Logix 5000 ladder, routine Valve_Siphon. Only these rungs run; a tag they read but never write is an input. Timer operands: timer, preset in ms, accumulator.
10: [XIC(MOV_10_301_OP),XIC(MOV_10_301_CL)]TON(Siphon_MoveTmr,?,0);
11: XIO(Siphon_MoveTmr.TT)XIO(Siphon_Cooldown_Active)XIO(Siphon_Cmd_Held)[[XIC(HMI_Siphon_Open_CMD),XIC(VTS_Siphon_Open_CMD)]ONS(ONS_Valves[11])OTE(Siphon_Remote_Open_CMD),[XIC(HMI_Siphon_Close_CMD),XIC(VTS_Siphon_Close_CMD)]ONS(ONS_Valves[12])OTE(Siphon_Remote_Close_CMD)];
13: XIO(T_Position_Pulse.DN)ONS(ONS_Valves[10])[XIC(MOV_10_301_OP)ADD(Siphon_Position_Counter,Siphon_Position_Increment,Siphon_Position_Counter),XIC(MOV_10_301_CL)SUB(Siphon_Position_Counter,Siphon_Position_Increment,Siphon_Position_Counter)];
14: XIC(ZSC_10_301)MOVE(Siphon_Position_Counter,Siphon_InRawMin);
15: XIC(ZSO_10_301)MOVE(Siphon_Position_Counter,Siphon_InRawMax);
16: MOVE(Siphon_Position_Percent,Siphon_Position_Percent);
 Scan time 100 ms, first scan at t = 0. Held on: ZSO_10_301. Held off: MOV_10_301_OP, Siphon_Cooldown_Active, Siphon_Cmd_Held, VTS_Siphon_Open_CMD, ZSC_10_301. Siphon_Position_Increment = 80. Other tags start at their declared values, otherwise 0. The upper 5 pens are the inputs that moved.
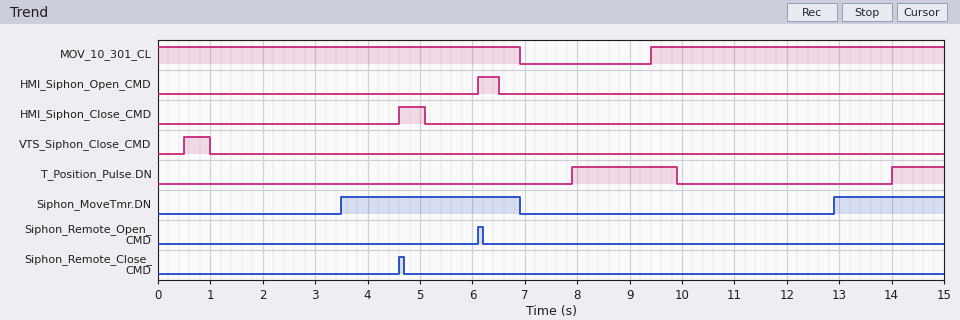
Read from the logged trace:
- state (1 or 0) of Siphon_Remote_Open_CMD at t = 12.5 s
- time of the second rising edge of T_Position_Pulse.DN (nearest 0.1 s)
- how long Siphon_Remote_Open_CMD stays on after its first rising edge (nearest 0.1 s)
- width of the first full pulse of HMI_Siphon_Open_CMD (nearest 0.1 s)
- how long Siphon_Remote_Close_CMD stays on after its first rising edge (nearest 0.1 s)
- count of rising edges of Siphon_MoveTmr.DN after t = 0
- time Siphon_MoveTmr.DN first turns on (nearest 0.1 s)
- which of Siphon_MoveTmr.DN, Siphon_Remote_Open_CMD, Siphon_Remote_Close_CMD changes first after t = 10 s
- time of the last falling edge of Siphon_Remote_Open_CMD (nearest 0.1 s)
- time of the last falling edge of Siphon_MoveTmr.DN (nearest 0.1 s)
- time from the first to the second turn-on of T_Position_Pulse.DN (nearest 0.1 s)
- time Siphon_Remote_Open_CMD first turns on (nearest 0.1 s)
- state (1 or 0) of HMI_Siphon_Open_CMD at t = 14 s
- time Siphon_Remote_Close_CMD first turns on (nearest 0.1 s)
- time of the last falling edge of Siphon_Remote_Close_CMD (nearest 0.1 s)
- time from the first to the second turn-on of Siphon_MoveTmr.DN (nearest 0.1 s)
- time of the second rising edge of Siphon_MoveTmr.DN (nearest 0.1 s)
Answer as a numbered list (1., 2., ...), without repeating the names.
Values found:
1. 0
2. 14.0 s
3. 0.1 s
4. 0.4 s
5. 0.1 s
6. 2
7. 3.5 s
8. Siphon_MoveTmr.DN
9. 6.2 s
10. 6.9 s
11. 6.1 s
12. 6.1 s
13. 0
14. 4.6 s
15. 4.7 s
16. 9.4 s
17. 12.9 s
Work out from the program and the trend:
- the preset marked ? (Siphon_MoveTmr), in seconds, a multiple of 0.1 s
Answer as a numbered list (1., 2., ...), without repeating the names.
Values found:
1. 3.5 s
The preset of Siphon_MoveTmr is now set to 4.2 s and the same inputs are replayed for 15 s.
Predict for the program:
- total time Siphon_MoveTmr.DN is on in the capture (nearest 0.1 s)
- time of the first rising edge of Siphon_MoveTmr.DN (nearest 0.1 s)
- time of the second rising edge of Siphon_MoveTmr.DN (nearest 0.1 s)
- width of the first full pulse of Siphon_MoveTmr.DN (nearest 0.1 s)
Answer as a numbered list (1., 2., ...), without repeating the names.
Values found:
1. 4.1 s
2. 4.2 s
3. 13.6 s
4. 2.7 s
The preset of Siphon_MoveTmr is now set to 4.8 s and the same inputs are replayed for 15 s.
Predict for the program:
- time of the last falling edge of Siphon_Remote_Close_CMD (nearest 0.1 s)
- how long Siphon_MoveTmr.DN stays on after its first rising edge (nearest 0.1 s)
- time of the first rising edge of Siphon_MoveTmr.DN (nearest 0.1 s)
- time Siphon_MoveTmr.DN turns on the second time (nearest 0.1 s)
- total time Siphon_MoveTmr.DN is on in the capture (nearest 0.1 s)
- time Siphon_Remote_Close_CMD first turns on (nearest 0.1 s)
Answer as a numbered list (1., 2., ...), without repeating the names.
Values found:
1. 4.9 s
2. 2.1 s
3. 4.8 s
4. 14.2 s
5. 2.9 s
6. 4.8 s
